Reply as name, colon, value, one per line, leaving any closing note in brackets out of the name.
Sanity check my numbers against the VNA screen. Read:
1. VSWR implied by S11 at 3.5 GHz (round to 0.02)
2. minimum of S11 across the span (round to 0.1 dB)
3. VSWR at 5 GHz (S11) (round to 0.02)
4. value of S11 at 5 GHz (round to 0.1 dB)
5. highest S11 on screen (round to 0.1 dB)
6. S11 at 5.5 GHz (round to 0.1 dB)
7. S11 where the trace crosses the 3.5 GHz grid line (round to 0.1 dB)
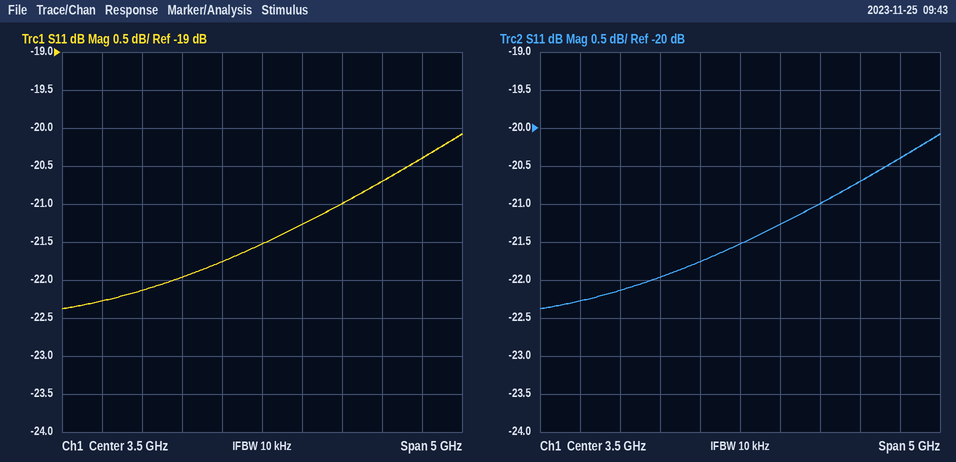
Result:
VSWR implied by S11 at 3.5 GHz: 1.18
minimum of S11 across the span: -22.4 dB
VSWR at 5 GHz (S11): 1.20
value of S11 at 5 GHz: -20.7 dB
highest S11 on screen: -20.1 dB
S11 at 5.5 GHz: -20.4 dB
S11 where the trace crosses the 3.5 GHz grid line: -21.5 dB
